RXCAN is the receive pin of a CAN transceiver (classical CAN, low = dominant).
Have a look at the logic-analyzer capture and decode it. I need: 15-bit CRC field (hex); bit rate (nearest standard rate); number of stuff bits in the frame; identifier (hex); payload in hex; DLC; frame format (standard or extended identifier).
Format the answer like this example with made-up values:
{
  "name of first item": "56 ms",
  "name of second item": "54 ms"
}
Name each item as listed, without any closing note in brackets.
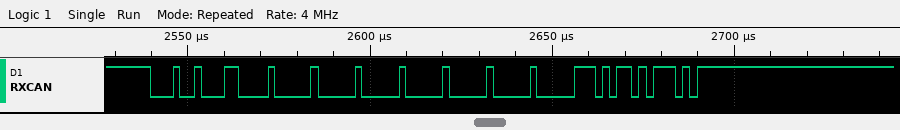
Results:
{
  "15-bit CRC field": "0x35AE",
  "bit rate": "500 kbit/s",
  "number of stuff bits in the frame": "7",
  "identifier": "0x123",
  "payload in hex": "00 00 00 00",
  "DLC": "4",
  "frame format": "standard"
}
